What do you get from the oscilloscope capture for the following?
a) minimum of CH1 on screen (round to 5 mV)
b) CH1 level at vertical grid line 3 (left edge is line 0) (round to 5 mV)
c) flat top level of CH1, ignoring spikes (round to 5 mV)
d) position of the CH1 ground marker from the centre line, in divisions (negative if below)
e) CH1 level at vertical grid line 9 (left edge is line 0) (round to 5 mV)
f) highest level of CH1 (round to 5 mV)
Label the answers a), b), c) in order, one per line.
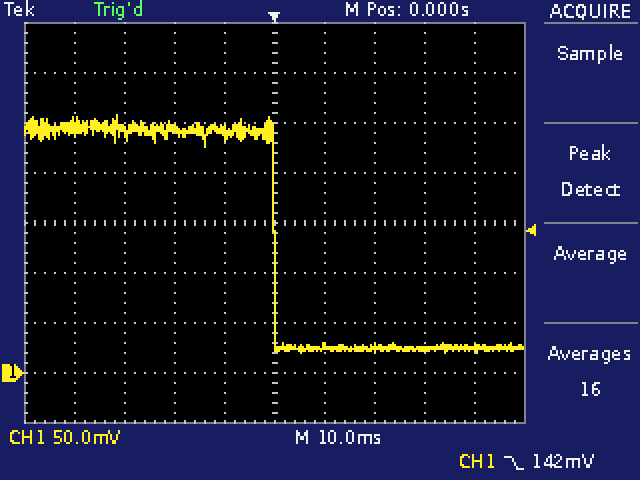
a) 20 mV
b) 245 mV
c) 245 mV
d) -3.0 div
e) 25 mV
f) 260 mV
